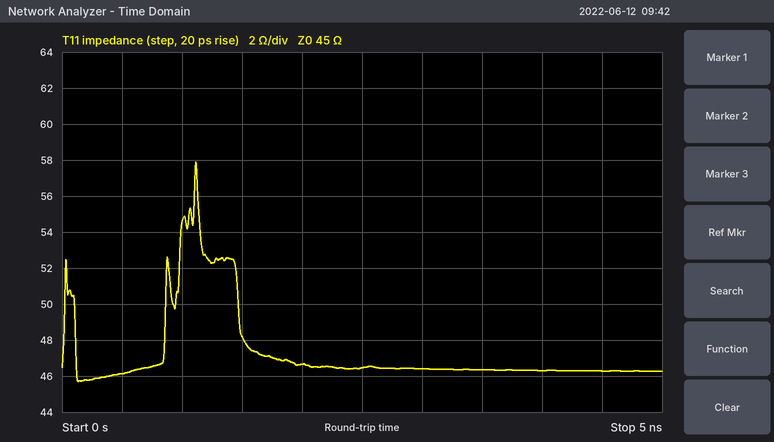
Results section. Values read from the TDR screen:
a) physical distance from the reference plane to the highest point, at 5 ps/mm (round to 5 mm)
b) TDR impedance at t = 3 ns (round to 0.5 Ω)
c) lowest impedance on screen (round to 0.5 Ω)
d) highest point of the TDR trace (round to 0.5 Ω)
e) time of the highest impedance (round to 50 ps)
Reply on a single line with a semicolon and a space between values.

110 mm; 46.5 Ω; 45.5 Ω; 58.0 Ω; 1.10 ns
